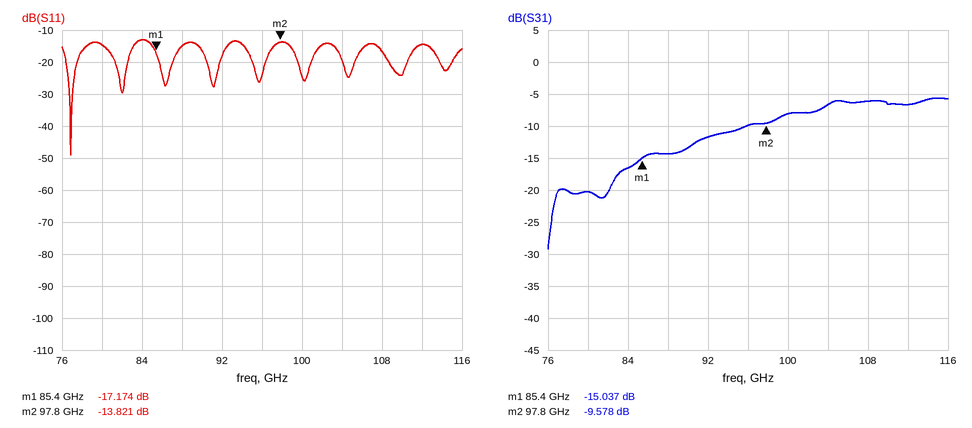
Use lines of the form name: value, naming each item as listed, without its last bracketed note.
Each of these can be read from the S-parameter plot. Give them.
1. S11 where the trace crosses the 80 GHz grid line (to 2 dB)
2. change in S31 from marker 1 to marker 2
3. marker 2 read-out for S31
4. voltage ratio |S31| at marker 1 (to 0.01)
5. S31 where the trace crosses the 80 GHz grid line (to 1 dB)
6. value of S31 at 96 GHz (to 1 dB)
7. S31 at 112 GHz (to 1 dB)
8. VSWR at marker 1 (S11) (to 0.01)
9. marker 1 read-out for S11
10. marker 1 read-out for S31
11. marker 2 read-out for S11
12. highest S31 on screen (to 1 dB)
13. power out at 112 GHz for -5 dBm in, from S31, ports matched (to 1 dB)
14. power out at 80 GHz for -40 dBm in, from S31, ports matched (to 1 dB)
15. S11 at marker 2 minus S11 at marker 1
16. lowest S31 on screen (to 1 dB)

S11 where the trace crosses the 80 GHz grid line: -14 dB
change in S31 from marker 1 to marker 2: 5.459 dB
marker 2 read-out for S31: -9.578 dB
voltage ratio |S31| at marker 1: 0.18
S31 where the trace crosses the 80 GHz grid line: -20 dB
value of S31 at 96 GHz: -10 dB
S31 at 112 GHz: -7 dB
VSWR at marker 1 (S11): 1.32
marker 1 read-out for S11: -17.174 dB
marker 1 read-out for S31: -15.037 dB
marker 2 read-out for S11: -13.821 dB
highest S31 on screen: -6 dB
power out at 112 GHz for -5 dBm in, from S31, ports matched: -12 dBm
power out at 80 GHz for -40 dBm in, from S31, ports matched: -60 dBm
S11 at marker 2 minus S11 at marker 1: 3.353 dB
lowest S31 on screen: -29 dB
